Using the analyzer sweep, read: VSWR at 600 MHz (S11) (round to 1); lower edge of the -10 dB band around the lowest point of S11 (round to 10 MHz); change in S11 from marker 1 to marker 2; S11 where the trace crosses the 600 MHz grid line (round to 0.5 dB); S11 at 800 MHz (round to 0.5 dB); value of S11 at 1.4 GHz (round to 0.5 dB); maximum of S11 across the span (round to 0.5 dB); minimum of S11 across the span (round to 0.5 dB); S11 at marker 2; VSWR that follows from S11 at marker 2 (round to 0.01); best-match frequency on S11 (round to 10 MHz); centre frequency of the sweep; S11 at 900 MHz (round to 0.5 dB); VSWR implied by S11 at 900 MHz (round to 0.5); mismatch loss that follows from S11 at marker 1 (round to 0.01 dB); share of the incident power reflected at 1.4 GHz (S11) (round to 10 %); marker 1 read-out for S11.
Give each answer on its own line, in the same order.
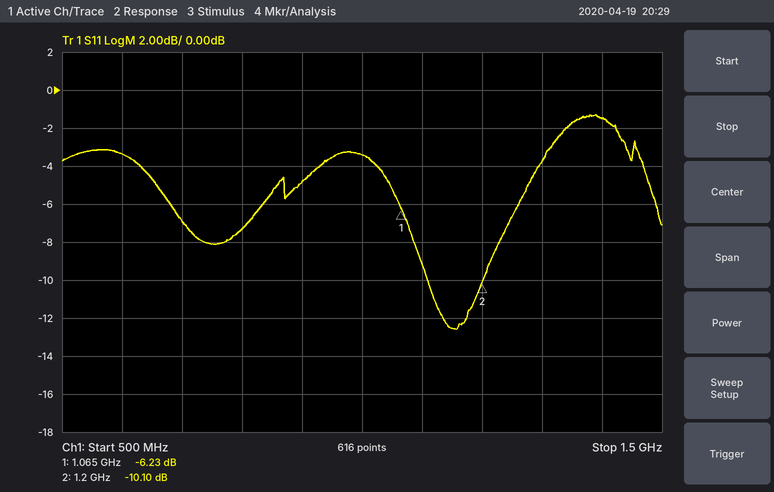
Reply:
5
1.11 GHz
-3.87 dB
-3.5 dB
-7.5 dB
-1.5 dB
-1.5 dB
-12.5 dB
-10.10 dB
1.91
1.16 GHz
1 GHz
-5.0 dB
3.5
1.18 dB
70 %
-6.23 dB
